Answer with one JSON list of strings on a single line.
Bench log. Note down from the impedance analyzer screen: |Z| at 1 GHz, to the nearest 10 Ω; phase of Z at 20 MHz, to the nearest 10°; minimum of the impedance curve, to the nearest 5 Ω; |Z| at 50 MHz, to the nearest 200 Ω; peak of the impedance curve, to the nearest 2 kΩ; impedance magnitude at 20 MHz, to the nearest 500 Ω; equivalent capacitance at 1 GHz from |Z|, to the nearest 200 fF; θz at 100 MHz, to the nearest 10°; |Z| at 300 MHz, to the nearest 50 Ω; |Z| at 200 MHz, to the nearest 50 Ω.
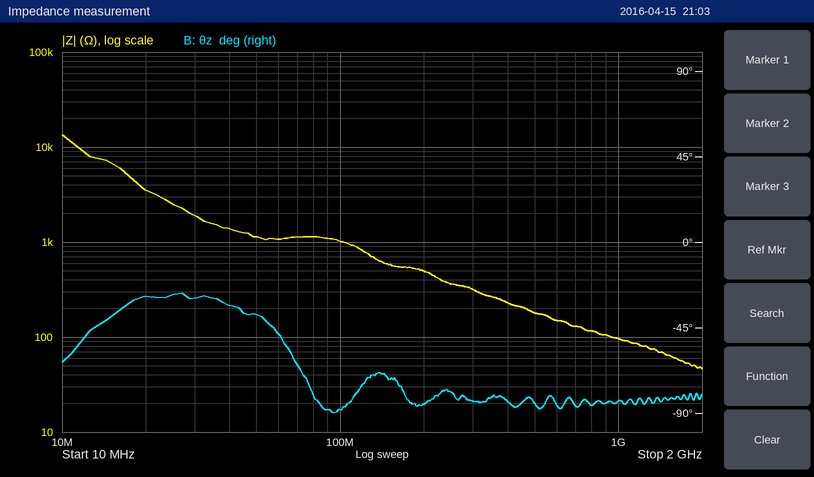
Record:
["100 Ω", "-30°", "45 Ω", "1.2 kΩ", "14 kΩ", "3.5 kΩ", "1.6 pF", "-90°", "300 Ω", "500 Ω"]
